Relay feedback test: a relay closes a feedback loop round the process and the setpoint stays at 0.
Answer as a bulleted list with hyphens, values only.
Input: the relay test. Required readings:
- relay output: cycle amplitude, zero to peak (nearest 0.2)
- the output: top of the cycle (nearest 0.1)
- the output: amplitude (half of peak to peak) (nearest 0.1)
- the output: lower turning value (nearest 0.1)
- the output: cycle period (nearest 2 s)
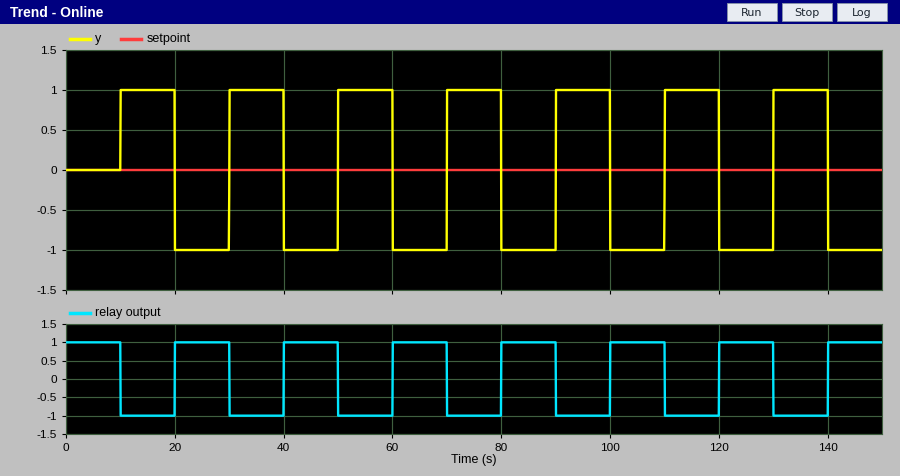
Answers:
- 1.0
- 1.0
- 1.0
- -1.0
- 20 s
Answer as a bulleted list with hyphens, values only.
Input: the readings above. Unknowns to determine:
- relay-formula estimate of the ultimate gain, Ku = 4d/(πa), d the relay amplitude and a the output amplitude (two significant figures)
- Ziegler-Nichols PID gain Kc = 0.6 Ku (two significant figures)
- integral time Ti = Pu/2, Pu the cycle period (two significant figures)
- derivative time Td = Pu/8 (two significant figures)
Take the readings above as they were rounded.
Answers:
- 1.3
- 0.78
- 10 s
- 2.5 s
